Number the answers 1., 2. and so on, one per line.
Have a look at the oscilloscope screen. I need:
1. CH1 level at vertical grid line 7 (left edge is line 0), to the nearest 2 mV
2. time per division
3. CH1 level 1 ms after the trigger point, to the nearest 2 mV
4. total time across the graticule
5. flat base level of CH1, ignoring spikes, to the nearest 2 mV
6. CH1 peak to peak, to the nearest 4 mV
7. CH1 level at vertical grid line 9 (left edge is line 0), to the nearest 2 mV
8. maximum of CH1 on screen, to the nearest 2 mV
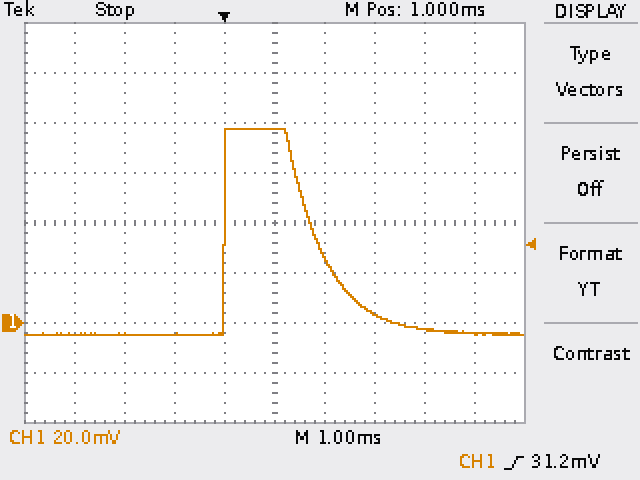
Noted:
1. 4 mV
2. 1 ms
3. 78 mV
4. 10 ms
5. -4 mV
6. 84 mV
7. -4 mV
8. 78 mV
